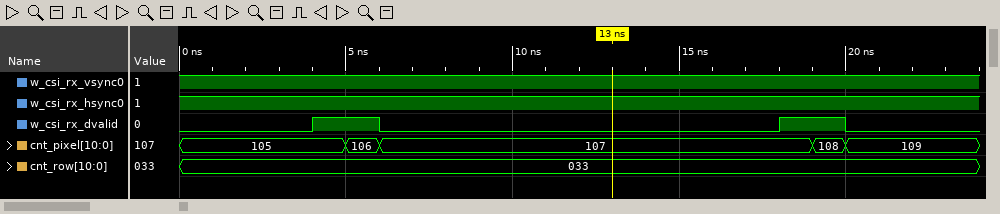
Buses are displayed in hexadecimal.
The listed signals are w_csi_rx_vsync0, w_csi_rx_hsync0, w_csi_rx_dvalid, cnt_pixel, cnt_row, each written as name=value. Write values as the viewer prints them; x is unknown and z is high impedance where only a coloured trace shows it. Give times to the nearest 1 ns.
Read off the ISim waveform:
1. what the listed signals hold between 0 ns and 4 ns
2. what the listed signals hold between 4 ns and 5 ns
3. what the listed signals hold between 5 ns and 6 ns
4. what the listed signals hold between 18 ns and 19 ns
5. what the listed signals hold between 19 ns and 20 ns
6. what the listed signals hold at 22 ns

w_csi_rx_vsync0=1, w_csi_rx_hsync0=1, w_csi_rx_dvalid=0, cnt_pixel=105, cnt_row=033
w_csi_rx_vsync0=1, w_csi_rx_hsync0=1, w_csi_rx_dvalid=1, cnt_pixel=105, cnt_row=033
w_csi_rx_vsync0=1, w_csi_rx_hsync0=1, w_csi_rx_dvalid=1, cnt_pixel=106, cnt_row=033
w_csi_rx_vsync0=1, w_csi_rx_hsync0=1, w_csi_rx_dvalid=1, cnt_pixel=107, cnt_row=033
w_csi_rx_vsync0=1, w_csi_rx_hsync0=1, w_csi_rx_dvalid=1, cnt_pixel=108, cnt_row=033
w_csi_rx_vsync0=1, w_csi_rx_hsync0=1, w_csi_rx_dvalid=0, cnt_pixel=109, cnt_row=033
